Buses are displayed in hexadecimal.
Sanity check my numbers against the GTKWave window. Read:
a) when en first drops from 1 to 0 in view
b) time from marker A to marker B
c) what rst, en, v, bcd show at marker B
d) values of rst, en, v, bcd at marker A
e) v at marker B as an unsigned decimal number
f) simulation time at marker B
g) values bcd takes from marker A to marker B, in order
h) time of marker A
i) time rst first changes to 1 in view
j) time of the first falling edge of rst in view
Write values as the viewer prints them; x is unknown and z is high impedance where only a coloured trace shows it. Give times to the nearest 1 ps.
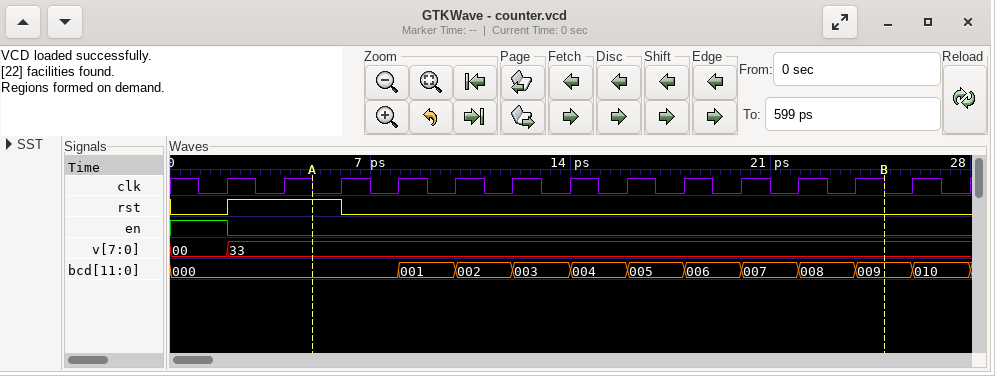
2 ps
20 ps
rst=0, en=0, v=33, bcd=009
rst=1, en=0, v=33, bcd=000
51
25 ps
000, 001, 002, 003, 004, 005, 006, 007, 008, 009
5 ps
2 ps
6 ps
